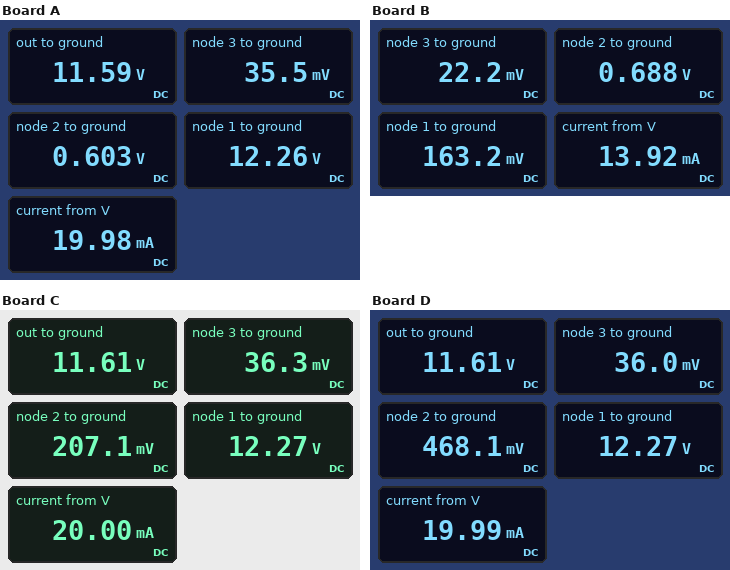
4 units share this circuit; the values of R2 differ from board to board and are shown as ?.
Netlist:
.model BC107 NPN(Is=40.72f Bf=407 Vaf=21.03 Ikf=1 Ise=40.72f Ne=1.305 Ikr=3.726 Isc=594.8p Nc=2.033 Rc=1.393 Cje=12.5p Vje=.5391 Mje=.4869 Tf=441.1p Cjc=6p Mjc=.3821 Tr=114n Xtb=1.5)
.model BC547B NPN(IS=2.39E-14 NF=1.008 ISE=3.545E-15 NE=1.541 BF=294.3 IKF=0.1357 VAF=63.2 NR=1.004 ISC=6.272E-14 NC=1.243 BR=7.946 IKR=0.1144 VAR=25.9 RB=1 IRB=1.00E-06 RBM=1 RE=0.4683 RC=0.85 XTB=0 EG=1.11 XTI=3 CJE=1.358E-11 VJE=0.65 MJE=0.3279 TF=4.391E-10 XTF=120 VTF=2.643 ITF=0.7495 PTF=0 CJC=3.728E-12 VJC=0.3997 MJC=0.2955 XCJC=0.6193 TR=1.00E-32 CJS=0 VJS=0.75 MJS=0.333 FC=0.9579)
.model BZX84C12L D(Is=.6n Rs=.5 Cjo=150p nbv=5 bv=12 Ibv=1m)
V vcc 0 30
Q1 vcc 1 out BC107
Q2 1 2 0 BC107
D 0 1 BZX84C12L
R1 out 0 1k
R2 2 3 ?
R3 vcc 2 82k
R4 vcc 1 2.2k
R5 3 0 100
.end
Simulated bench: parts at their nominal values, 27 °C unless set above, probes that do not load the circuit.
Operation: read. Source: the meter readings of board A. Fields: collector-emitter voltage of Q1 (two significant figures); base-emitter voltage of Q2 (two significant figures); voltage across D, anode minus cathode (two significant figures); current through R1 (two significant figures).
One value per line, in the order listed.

18 V
600 mV
-12 V
12 mA
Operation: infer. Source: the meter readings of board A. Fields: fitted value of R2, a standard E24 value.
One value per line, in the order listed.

1.6 kΩ
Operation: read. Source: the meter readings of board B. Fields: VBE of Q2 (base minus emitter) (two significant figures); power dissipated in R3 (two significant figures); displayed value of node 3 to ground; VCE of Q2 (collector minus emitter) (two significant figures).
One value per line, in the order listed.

690 mV
10 mW
22.2 mV
160 mV
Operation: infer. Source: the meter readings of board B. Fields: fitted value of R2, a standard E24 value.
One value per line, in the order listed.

3 kΩ
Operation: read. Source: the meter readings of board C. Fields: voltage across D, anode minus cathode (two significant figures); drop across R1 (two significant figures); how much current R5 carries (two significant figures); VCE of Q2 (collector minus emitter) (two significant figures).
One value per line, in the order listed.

-12 V
12 V
360 µA
12 V
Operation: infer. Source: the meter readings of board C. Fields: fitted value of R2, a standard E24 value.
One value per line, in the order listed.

470 Ω
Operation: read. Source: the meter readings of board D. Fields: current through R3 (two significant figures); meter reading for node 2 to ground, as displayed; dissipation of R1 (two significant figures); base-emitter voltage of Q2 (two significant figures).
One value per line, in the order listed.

360 µA
468.1 mV
130 mW
470 mV
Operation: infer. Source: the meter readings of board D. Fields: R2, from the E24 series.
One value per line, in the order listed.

1.2 kΩ
